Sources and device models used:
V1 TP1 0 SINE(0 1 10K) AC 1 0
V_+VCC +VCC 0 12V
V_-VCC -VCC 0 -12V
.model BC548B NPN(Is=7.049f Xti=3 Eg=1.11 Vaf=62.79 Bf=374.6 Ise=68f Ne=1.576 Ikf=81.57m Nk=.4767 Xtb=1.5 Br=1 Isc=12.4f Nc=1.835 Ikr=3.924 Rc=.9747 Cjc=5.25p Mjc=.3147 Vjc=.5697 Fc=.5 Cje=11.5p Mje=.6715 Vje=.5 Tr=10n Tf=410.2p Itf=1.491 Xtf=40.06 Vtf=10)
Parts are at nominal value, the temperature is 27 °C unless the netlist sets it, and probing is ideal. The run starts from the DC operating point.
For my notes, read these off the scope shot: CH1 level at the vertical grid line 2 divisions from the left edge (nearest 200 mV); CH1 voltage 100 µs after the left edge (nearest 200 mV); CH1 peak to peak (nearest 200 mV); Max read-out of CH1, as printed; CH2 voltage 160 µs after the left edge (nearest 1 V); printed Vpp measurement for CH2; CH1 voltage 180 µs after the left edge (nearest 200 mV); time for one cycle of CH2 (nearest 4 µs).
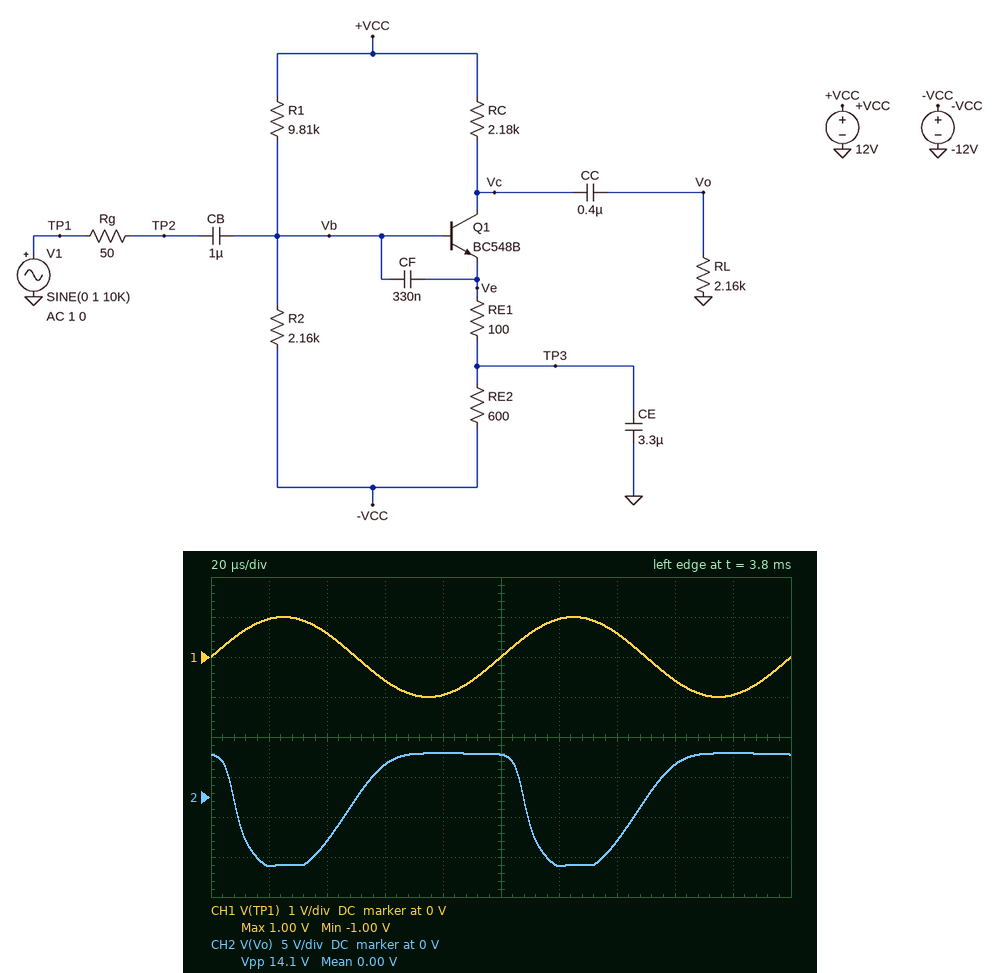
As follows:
600 mV
0 V
2.0 V
1.00 V
4 V
14.1 V
-1.0 V
100 µs
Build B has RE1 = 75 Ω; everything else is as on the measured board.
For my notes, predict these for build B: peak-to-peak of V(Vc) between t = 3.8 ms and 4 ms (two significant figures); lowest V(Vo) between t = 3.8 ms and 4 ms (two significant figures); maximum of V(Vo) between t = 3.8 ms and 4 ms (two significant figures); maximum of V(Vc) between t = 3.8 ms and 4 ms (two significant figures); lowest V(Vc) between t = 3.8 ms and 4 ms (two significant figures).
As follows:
15 V
-9.5 V
5.2 V
6.8 V
-7.8 V
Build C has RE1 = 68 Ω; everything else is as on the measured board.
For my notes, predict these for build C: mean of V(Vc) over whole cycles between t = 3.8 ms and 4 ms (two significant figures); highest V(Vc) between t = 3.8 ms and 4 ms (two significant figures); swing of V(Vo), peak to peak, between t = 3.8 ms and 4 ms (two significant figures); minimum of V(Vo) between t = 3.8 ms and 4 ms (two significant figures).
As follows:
1.8 V
6.9 V
15 V
-9.8 V
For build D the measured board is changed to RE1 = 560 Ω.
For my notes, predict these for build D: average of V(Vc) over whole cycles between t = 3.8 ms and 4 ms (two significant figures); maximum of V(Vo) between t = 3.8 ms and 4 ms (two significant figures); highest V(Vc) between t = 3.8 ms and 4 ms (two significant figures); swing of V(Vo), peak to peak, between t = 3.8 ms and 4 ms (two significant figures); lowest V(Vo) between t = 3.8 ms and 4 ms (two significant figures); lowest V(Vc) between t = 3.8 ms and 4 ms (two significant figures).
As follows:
5.2 V
1.7 V
6.9 V
3.6 V
-1.8 V
3.4 V
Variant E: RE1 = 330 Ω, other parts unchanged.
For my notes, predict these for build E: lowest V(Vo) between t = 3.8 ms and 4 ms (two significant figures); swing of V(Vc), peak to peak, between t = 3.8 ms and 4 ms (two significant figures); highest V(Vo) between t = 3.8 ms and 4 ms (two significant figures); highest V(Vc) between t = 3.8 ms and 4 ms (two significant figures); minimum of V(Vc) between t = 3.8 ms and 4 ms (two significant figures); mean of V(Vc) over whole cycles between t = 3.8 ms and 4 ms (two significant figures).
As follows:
-3.1 V
6.0 V
2.9 V
6.4 V
460 mV
3.5 V
